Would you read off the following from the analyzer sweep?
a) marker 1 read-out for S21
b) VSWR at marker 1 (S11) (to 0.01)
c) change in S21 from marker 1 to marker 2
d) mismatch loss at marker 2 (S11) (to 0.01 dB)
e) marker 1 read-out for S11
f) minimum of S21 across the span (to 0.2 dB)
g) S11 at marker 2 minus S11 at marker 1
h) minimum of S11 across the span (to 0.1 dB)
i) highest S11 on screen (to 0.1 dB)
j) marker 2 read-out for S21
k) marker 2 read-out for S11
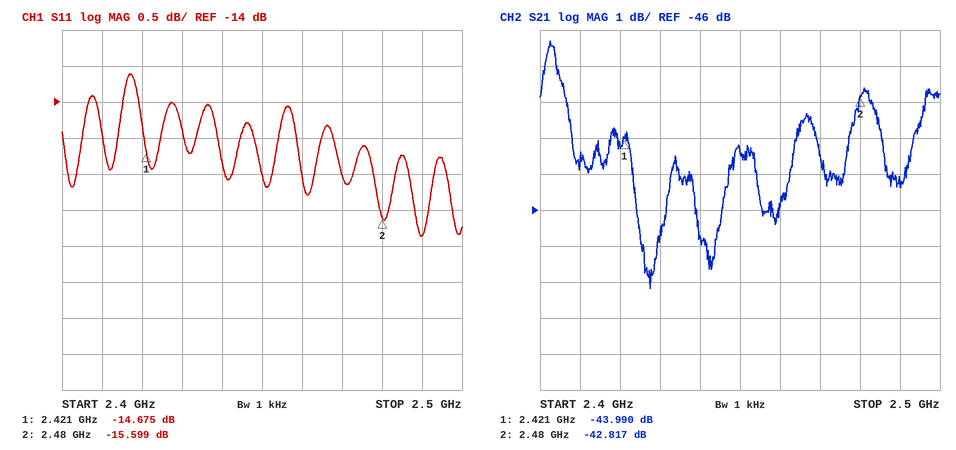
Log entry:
-43.990 dB
1.45
1.173 dB
0.12 dB
-14.675 dB
-48.2 dB
-0.924 dB
-15.9 dB
-13.6 dB
-42.817 dB
-15.599 dB
